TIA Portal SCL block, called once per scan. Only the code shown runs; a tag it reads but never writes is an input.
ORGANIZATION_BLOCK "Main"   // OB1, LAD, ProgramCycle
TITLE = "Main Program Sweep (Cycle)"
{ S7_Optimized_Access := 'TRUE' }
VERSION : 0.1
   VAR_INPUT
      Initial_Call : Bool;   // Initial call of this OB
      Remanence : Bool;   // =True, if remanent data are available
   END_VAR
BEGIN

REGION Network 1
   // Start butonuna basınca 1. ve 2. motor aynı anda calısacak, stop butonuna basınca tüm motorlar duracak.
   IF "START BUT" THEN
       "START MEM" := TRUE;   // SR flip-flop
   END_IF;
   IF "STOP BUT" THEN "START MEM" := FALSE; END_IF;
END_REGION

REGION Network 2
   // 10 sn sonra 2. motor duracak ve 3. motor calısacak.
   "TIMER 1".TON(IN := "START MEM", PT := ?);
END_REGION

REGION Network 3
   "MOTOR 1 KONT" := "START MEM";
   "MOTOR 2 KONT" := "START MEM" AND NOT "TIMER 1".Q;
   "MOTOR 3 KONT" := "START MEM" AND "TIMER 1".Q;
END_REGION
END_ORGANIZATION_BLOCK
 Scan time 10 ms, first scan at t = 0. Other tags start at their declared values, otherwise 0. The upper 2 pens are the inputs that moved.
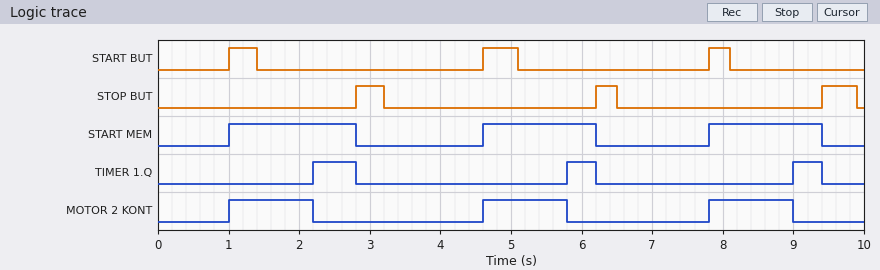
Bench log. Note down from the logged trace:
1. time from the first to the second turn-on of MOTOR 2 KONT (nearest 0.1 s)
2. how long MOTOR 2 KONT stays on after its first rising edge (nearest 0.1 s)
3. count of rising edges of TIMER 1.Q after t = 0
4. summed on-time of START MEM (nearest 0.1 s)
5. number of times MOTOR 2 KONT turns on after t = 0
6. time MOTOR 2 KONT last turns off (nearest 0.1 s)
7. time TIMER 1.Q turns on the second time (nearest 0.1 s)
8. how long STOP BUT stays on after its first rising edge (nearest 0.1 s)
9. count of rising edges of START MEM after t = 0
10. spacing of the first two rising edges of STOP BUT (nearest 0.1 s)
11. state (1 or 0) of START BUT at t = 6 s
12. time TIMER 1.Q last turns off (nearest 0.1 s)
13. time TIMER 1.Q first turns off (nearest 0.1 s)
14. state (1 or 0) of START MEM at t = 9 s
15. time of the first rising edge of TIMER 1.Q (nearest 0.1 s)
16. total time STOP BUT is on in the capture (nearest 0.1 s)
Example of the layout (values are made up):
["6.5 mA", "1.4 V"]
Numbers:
["3.6 s", "1.2 s", "3", "5.0 s", "3", "9.0 s", "5.8 s", "0.4 s", "3", "3.4 s", "0", "9.4 s", "2.8 s", "1", "2.2 s", "1.2 s"]
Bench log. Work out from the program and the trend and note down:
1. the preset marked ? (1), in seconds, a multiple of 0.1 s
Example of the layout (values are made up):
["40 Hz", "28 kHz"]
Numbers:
["1.2 s"]
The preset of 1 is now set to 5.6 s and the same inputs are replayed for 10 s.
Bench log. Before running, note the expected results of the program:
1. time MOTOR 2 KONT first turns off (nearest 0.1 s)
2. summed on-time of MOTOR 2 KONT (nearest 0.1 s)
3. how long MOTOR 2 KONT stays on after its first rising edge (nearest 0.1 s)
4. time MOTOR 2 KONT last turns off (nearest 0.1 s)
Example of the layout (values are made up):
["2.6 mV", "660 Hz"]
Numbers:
["2.8 s", "5.0 s", "1.8 s", "9.4 s"]
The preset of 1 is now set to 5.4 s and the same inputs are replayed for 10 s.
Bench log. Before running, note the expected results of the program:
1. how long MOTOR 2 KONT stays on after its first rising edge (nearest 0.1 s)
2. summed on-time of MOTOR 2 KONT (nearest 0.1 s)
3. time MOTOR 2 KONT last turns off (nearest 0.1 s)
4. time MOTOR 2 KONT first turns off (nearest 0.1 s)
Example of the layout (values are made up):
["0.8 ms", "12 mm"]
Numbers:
["1.8 s", "5.0 s", "9.4 s", "2.8 s"]
